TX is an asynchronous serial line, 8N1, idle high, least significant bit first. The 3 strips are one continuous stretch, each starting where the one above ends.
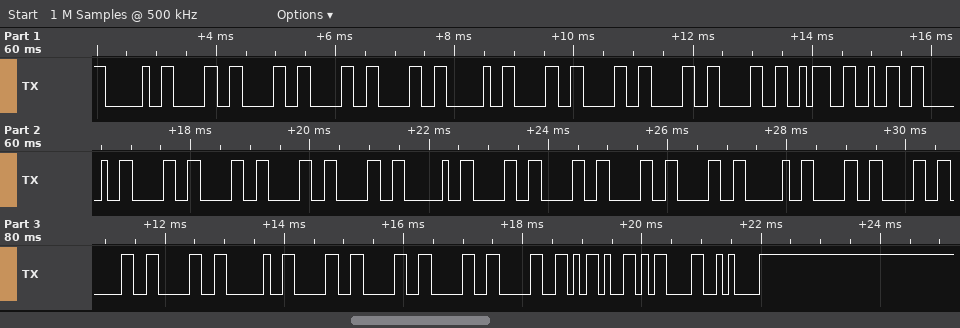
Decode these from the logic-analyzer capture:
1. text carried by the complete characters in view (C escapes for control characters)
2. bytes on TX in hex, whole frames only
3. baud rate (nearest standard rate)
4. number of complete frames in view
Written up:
" 0000 0000:2 0000 0000 0000 0000-\r\n"
0x20 0x30 0x30 0x30 0x30 0x20 0x30 0x30 0x30 0x30 0x3A 0x32 0x20 0x30 0x30 0x30 0x30 0x20 0x30 0x30 0x30 0x30 0x20 0x30 0x30 0x30 0x30 0x20 0x30 0x30 0x30 0x30 0x2D 0x0D 0x0A
9600 baud
35
